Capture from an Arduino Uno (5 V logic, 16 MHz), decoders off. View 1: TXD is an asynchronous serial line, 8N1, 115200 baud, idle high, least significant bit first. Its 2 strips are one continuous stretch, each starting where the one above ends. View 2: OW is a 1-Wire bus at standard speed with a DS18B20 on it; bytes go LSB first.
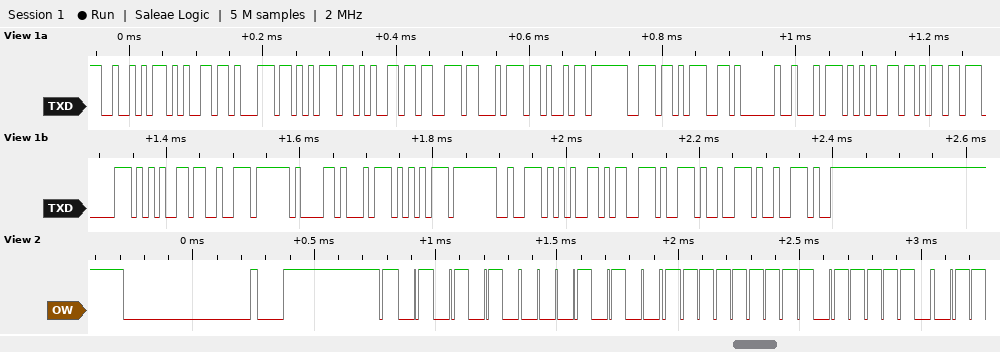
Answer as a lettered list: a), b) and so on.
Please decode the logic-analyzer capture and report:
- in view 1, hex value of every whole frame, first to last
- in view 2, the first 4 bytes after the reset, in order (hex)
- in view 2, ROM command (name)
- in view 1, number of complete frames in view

a) 52 65 71 75 65 73 74 69 6E 67 20 74 65 6D 70 65 72 61 74 75 72 65 73 2E 2E 2E
b) 55 28 FF 7D
c) Match ROM
d) 26
